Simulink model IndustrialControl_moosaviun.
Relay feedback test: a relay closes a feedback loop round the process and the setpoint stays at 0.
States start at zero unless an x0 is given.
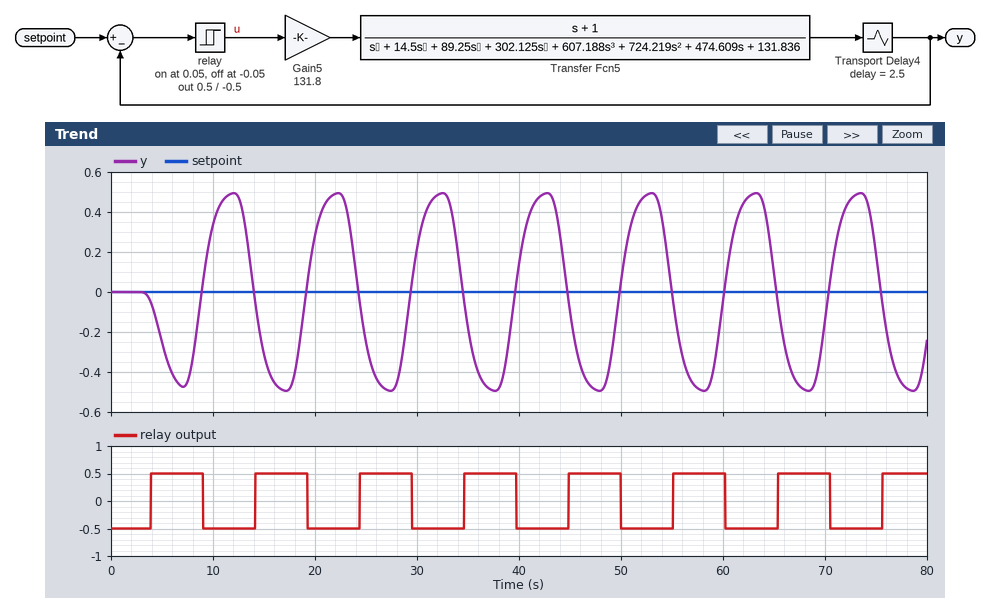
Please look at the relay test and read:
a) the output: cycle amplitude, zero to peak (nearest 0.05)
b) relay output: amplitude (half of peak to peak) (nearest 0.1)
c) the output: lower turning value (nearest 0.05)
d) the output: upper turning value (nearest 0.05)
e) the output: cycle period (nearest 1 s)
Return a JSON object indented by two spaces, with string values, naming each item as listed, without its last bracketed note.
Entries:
{
  "the output: cycle amplitude, zero to peak": "0.50",
  "relay output: amplitude (half of peak to peak)": "0.5",
  "the output: lower turning value": "-0.50",
  "the output: upper turning value": "0.50",
  "the output: cycle period": "10 s"
}
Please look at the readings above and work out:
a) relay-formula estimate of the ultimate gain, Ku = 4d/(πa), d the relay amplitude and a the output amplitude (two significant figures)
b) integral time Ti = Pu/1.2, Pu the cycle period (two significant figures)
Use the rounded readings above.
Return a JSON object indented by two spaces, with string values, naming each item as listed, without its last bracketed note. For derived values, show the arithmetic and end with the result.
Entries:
{
  "relay-formula estimate of the ultimate gain, Ku = 4d/(πa), d the relay amplitude and a the output amplitude": "4 × 0.5 / (π × 0.5) = 1.3",
  "integral time Ti = Pu/1.2, Pu the cycle period": "10 / 1.2 = 8.3 s"
}
